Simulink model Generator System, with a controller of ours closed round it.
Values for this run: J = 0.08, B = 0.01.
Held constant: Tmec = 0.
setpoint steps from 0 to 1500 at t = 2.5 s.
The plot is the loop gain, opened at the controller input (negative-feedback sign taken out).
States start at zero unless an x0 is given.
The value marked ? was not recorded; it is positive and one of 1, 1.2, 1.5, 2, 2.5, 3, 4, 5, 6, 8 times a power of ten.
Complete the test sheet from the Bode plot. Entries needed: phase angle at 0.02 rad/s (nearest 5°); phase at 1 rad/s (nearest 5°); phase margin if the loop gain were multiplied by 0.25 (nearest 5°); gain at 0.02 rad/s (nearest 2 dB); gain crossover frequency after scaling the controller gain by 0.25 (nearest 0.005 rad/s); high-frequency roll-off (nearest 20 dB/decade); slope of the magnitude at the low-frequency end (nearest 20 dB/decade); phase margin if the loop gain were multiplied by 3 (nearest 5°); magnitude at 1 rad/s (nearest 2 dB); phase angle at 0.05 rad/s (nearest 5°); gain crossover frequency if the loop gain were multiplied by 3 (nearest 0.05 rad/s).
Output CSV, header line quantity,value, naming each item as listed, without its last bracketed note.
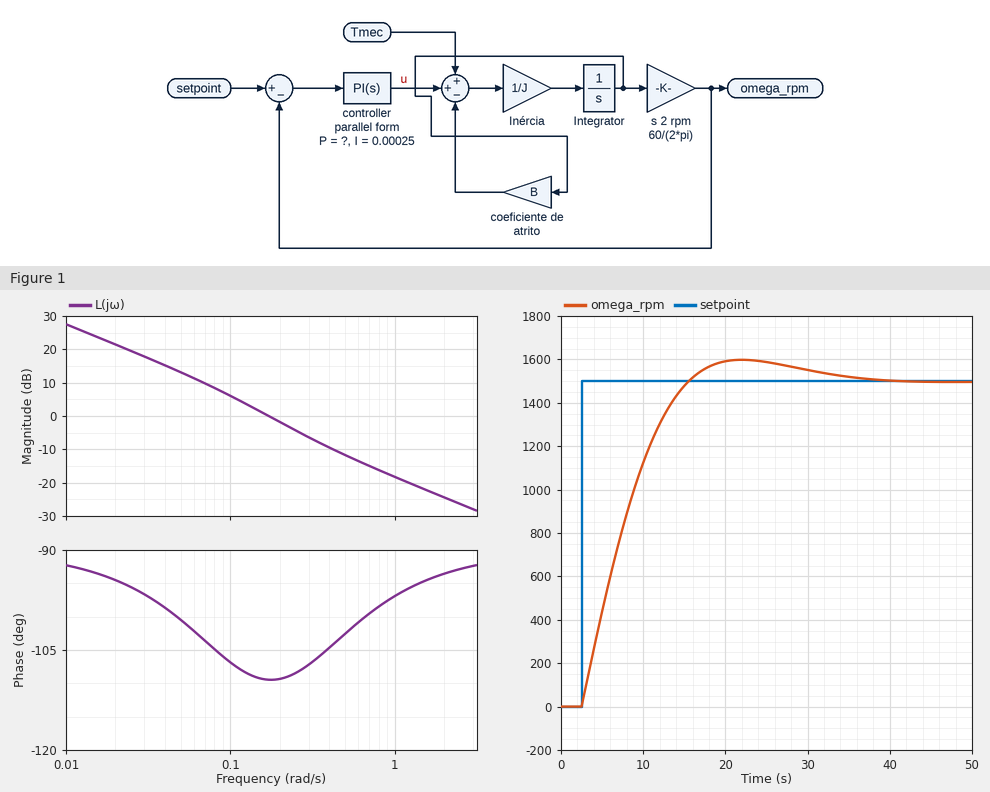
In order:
quantity,value
phase angle at 0.02 rad/s,-95°
phase at 1 rad/s,-95°
phase margin if the loop gain were multiplied by 0.25,80°
gain at 0.02 rad/s,22 dB
gain crossover frequency after scaling the controller gain by 0.25,0.055 rad/s
high-frequency roll-off,-20 dB/decade
slope of the magnitude at the low-frequency end,-20 dB/decade
phase margin if the loop gain were multiplied by 3,75°
magnitude at 1 rad/s,-18 dB
phase angle at 0.05 rad/s,-100°
gain crossover frequency if the loop gain were multiplied by 3,0.40 rad/s
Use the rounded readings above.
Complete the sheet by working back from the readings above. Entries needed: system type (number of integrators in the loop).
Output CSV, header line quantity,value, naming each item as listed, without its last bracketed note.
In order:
quantity,value
system type,1
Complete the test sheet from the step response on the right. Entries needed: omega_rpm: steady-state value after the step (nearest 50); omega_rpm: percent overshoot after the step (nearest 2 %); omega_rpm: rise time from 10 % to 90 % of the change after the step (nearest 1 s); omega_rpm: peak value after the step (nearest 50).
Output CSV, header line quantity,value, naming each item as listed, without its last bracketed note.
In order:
quantity,value
omega_rpm: steady-state value after the step,1500
omega_rpm: percent overshoot after the step,6 %
omega_rpm: rise time from 10 % to 90 % of the change after the step,9 s
omega_rpm: peak value after the step,1600
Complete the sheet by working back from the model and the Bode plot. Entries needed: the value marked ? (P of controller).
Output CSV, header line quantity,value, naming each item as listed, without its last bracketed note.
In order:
quantity,value
the value marked ?,0.001
